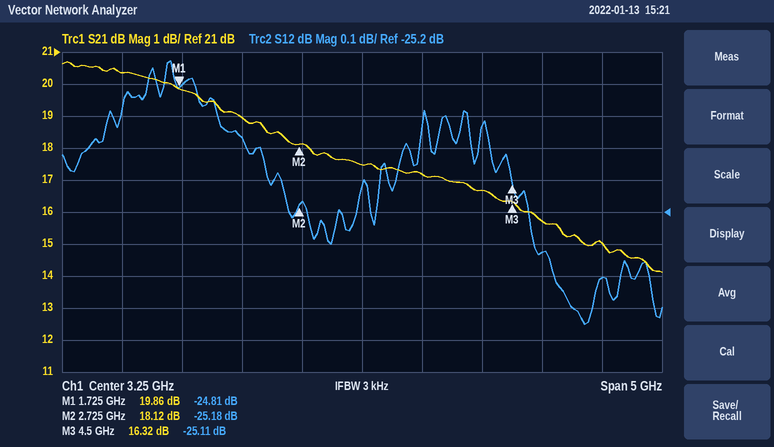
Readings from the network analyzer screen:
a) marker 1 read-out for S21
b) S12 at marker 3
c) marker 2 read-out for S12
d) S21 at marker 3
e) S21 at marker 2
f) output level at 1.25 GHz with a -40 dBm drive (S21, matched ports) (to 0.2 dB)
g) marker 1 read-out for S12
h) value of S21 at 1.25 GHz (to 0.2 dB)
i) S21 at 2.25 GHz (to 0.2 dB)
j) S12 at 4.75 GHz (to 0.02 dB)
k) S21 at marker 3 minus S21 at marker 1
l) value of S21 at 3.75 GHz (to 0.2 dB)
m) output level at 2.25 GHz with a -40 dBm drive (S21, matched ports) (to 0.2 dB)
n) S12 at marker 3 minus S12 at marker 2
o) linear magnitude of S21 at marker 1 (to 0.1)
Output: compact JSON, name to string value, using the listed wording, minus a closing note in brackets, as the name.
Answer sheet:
{"marker 1 read-out for S21": "19.86 dB", "S12 at marker 3": "-25.11 dB", "marker 2 read-out for S12": "-25.18 dB", "S21 at marker 3": "16.32 dB", "S21 at marker 2": "18.12 dB", "output level at 1.25 GHz with a -40 dBm drive (S21, matched ports)": "-19.6 dBm", "marker 1 read-out for S12": "-24.81 dB", "value of S21 at 1.25 GHz": "20.4 dB", "S21 at 2.25 GHz": "19.0 dB", "S12 at 4.75 GHz": "-25.32 dB", "S21 at marker 3 minus S21 at marker 1": "-3.54 dB", "value of S21 at 3.75 GHz": "17.2 dB", "output level at 2.25 GHz with a -40 dBm drive (S21, matched ports)": "-21.0 dBm", "S12 at marker 3 minus S12 at marker 2": "0.07 dB", "linear magnitude of S21 at marker 1": "9.8"}
